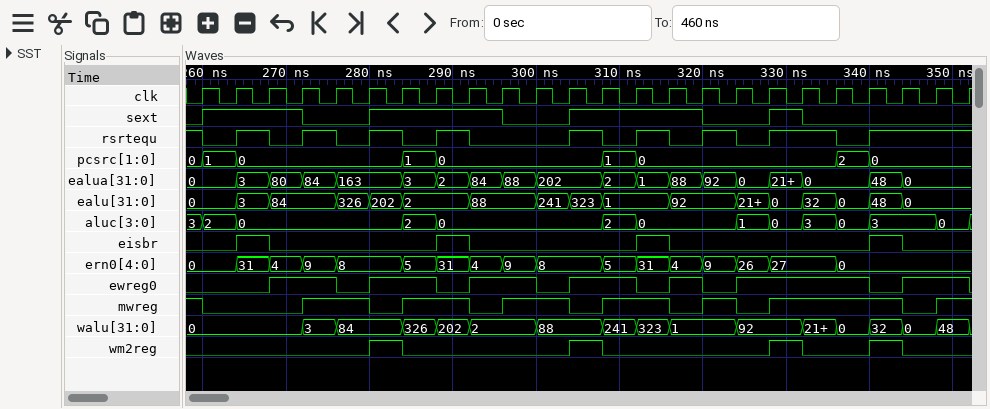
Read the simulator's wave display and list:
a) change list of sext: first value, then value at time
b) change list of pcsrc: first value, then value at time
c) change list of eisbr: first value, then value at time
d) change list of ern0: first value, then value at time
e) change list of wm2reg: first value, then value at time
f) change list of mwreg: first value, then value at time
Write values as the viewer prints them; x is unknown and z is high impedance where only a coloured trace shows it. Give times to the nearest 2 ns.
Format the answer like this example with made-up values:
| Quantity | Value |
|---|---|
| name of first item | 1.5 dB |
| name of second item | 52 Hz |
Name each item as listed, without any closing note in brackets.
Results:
| Quantity | Value |
|---|---|
| change list of sext: first value, then value at time | 0, 1 at 260 ns, 0 at 272 ns, 1 at 280 ns, 0 at 296 ns, 1 at 304 ns, 0 at 320 ns, 1 at 328 ns, 0 at 332 ns |
| change list of pcsrc: first value, then value at time | 0, 1 at 260 ns, 0 at 264 ns, 1 at 284 ns, 0 at 288 ns, 1 at 308 ns, 0 at 312 ns, 2 at 336 ns, 0 at 340 ns |
| change list of eisbr: first value, then value at time | 0, 1 at 264 ns, 0 at 268 ns, 1 at 288 ns, 0 at 292 ns, 1 at 312 ns, 0 at 316 ns, 1 at 340 ns, 0 at 344 ns |
| change list of ern0: first value, then value at time | 0, 31 at 264 ns, 4 at 268 ns, 9 at 272 ns, 8 at 276 ns, 5 at 284 ns, 31 at 288 ns, 4 at 292 ns, 9 at 296 ns, 8 at 300 ns, 5 at 308 ns, 31 at 312 ns, 4 at 316 ns, 9 at 320 ns, 26 at 324 ns, 27 at 328 ns, 0 at 336 ns |
| change list of wm2reg: first value, then value at time | 0, 1 at 280 ns, 0 at 284 ns, 1 at 304 ns, 0 at 308 ns, 1 at 328 ns, 0 at 332 ns, 1 at 340 ns, 0 at 344 ns |
| change list of mwreg: first value, then value at time | 1, 0 at 260 ns, 1 at 272 ns, 0 at 280 ns, 1 at 284 ns, 0 at 292 ns, 1 at 296 ns, 0 at 304 ns, 1 at 308 ns, 0 at 316 ns, 1 at 320 ns, 0 at 324 ns, 1 at 328 ns, 0 at 344 ns, 1 at 348 ns |
